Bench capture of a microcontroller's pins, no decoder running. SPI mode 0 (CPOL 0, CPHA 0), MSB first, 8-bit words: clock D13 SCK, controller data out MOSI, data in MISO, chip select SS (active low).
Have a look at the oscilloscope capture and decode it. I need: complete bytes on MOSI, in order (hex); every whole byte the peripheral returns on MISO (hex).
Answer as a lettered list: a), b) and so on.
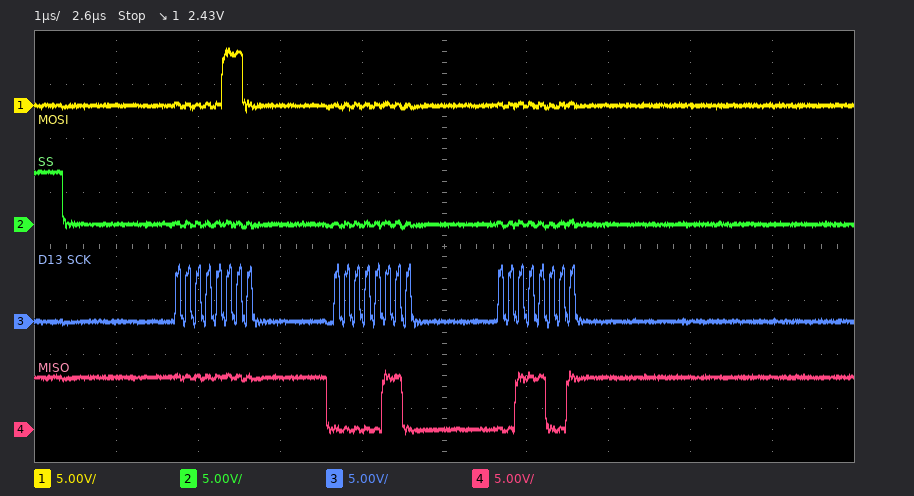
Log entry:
a) 06 00 00
b) FF 06 39
